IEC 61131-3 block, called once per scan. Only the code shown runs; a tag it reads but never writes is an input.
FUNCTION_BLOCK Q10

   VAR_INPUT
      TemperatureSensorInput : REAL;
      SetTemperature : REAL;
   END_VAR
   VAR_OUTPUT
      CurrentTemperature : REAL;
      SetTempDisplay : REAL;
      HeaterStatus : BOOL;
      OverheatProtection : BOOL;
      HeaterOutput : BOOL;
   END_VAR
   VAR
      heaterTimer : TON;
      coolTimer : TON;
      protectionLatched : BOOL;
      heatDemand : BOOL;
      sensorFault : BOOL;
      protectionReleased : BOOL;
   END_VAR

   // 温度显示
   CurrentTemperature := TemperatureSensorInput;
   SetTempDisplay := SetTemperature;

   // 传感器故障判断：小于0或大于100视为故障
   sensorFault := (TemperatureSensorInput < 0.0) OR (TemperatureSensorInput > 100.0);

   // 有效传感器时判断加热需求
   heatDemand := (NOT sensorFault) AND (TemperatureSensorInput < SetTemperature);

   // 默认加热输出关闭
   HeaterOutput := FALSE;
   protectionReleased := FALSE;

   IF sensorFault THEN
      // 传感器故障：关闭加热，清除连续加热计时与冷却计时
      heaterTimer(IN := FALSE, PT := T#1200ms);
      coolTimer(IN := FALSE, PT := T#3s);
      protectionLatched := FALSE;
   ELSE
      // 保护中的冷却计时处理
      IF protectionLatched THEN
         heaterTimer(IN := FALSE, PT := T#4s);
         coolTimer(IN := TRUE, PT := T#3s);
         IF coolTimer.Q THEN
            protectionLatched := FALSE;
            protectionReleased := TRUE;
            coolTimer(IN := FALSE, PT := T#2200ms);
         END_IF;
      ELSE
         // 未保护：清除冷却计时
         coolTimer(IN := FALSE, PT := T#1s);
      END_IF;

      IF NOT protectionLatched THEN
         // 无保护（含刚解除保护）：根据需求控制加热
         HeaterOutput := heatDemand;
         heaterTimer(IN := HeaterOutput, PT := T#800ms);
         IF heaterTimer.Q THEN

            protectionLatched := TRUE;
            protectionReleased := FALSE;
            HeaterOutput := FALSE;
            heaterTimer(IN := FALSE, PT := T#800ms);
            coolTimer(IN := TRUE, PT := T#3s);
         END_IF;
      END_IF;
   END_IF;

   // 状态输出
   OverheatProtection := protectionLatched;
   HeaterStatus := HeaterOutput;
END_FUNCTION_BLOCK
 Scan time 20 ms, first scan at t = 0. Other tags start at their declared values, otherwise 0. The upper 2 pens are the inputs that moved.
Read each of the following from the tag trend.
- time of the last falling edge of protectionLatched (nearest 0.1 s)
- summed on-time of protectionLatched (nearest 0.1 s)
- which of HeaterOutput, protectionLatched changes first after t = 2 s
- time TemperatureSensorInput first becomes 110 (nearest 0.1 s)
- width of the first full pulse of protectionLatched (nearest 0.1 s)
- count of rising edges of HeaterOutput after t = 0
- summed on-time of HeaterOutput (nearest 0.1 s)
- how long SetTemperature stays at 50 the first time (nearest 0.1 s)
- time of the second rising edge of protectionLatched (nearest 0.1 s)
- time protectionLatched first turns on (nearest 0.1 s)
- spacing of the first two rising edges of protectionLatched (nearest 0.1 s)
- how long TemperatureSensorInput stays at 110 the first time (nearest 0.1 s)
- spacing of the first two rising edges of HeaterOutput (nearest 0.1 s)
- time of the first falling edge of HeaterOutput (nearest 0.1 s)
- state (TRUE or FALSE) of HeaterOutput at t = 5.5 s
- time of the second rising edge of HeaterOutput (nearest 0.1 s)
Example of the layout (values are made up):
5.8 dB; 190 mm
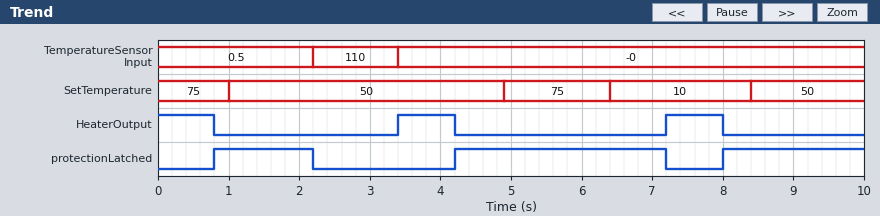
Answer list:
7.2 s; 6.4 s; protectionLatched; 2.2 s; 1.4 s; 2; 2.4 s; 3.9 s; 4.2 s; 0.8 s; 3.4 s; 1.2 s; 3.8 s; 0.8 s; FALSE; 7.2 s
